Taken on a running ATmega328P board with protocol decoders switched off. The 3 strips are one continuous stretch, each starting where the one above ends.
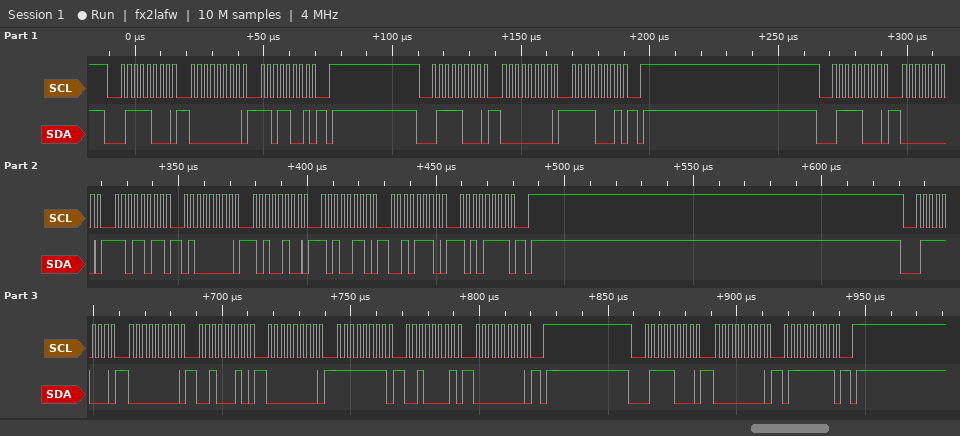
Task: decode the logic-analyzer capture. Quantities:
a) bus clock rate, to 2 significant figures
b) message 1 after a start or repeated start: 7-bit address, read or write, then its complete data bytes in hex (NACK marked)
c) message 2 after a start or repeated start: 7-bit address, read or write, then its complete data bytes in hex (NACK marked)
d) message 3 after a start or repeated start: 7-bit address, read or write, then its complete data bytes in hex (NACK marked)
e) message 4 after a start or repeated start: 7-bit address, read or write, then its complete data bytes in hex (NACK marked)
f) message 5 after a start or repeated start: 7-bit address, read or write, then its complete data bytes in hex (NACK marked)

400 kHz
0x3C write: 00 D9
0x3C write: 00 F1
0x3C write: 00 DB 40 A4 A6 2E AF
0x3C write: 00 22 00 FF 21 00
0x3C write: 00 7F
